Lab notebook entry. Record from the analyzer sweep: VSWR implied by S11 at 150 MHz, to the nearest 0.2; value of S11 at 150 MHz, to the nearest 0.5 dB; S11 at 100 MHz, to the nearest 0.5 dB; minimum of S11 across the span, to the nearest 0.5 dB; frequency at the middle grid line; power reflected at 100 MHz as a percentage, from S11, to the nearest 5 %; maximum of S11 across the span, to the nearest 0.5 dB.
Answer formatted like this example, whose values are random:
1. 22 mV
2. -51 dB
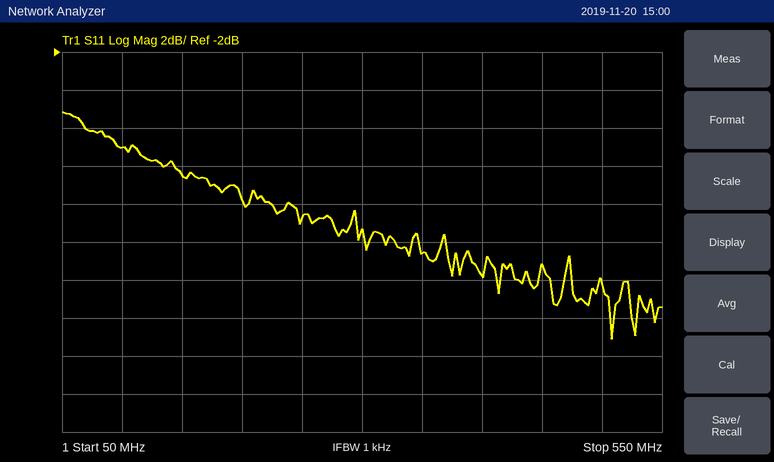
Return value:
1. 2.2
2. -8.5 dB
3. -7.0 dB
4. -17.0 dB
5. 300 MHz
6. 20 %
7. -5.0 dB
